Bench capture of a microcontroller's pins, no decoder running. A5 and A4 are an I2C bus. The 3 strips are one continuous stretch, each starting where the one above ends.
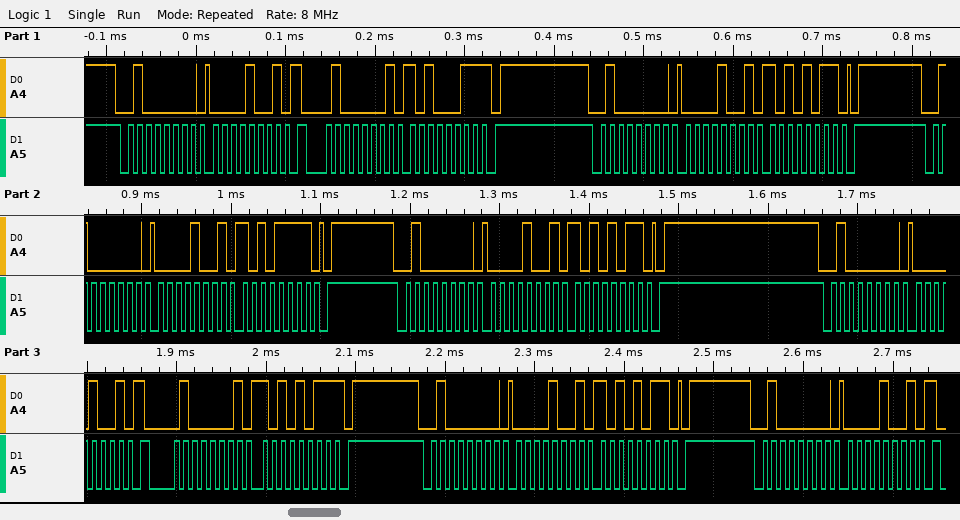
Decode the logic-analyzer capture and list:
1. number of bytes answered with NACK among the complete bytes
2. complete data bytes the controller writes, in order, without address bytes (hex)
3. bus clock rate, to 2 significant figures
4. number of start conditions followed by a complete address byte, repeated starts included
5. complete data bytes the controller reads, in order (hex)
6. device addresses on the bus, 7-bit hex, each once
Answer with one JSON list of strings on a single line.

["2", "09 09 AB 09 AF 09 AB 09 09 AB 09", "100 kHz", "9", "A3 AB", "0x20"]
